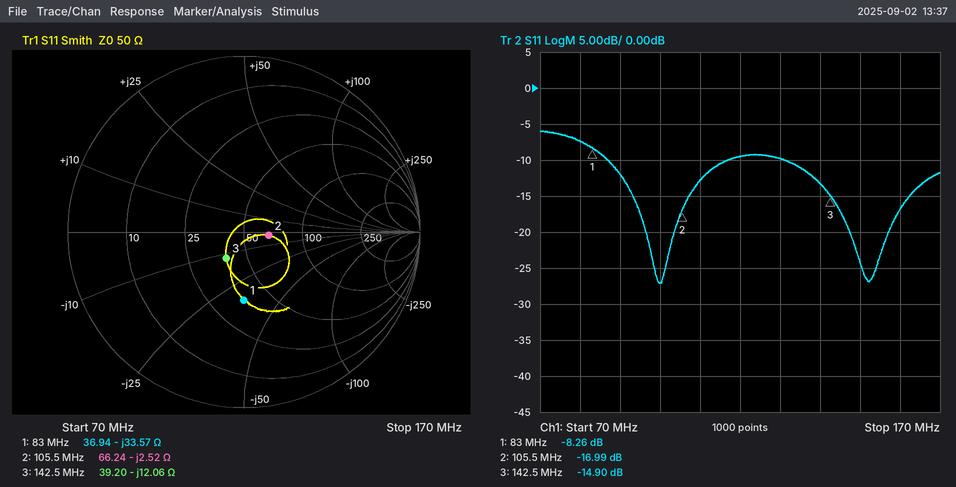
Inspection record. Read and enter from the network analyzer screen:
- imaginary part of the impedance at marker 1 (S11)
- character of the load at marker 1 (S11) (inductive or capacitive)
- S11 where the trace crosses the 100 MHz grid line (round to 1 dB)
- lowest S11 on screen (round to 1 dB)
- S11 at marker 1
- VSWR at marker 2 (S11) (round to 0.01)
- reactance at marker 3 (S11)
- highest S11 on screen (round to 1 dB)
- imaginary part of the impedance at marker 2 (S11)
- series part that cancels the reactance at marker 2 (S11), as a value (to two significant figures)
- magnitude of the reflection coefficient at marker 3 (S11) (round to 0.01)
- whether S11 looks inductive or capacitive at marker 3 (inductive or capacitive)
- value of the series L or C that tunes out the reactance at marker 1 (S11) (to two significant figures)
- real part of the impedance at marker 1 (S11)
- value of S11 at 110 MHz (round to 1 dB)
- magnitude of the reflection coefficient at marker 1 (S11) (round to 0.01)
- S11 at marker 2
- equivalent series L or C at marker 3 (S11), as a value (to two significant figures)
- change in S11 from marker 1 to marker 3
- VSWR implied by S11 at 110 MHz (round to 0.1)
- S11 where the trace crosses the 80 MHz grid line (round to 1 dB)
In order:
-33.57 Ω
capacitive
-27 dB
-27 dB
-8.26 dB
1.33
-12.06 Ω
-6 dB
-2.52 Ω
3.8 nH
0.18
capacitive
64 nH
36.94 Ω
-13 dB
0.39
-16.99 dB
93 pF
-6.64 dB
1.6
-7 dB
